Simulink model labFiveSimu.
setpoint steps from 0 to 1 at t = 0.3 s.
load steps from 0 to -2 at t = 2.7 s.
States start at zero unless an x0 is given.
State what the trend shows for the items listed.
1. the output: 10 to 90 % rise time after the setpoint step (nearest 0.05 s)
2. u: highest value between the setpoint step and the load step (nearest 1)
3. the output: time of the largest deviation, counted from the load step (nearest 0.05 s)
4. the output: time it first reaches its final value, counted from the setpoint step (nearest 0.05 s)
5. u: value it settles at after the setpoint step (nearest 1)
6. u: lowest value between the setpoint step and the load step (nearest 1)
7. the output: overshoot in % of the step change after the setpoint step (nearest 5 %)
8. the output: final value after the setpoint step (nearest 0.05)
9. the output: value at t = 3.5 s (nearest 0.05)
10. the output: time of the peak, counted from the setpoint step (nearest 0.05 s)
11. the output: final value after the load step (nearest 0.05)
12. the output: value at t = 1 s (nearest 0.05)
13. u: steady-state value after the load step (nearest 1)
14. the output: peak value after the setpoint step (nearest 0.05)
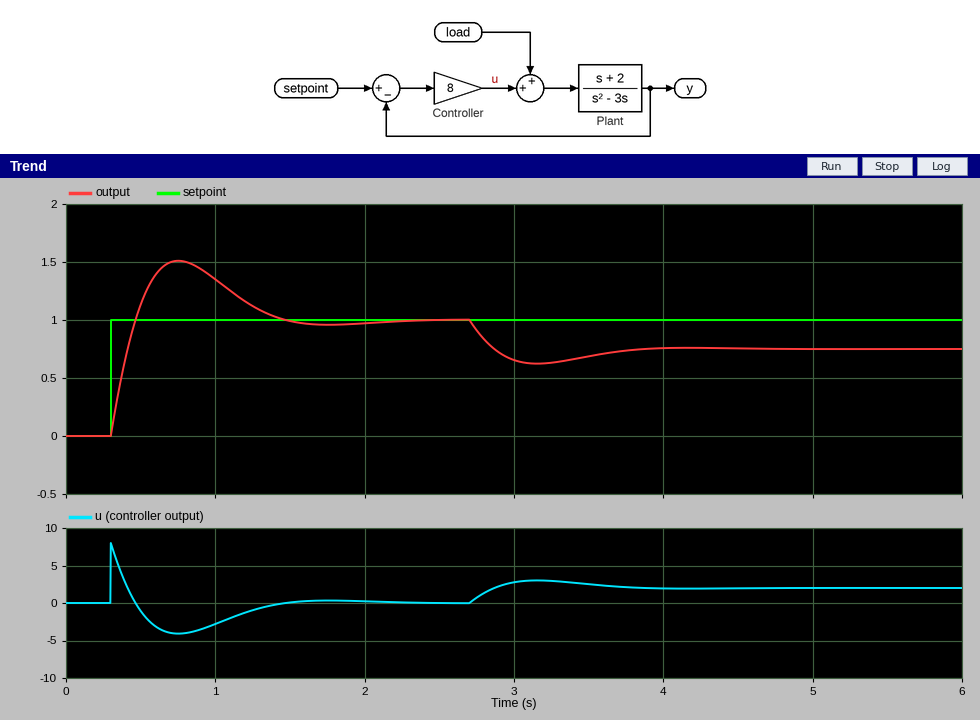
0.15 s
8
0.45 s
0.15 s
0
-4
50 %
1.00
0.70
0.45 s
0.75
1.35
2
1.50
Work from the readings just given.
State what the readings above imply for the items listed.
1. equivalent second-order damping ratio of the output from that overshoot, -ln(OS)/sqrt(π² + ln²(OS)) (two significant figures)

0.22
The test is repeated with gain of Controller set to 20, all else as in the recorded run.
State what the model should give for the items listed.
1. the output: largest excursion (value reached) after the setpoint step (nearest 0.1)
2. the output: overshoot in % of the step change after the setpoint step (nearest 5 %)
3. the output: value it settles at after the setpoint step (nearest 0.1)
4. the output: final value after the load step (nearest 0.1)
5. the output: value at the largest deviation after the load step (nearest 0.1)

1.2
20 %
1.0
0.9
0.9
